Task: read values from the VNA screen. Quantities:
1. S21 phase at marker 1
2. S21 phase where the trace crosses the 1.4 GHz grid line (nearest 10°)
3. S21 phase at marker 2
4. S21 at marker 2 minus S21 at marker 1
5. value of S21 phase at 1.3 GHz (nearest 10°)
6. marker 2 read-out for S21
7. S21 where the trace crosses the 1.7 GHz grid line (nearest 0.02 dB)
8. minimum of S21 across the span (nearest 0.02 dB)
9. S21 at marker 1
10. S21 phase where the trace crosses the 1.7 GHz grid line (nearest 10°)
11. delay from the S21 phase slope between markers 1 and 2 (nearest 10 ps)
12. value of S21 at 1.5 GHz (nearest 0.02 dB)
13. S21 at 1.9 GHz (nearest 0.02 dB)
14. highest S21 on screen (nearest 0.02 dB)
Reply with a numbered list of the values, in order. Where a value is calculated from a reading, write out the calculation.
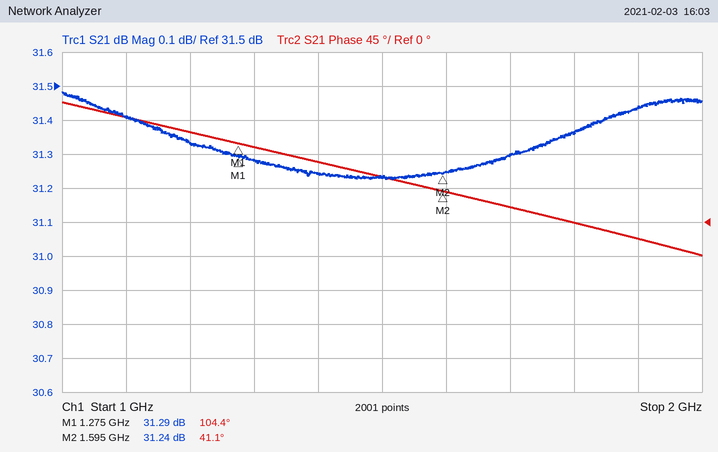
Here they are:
1. 104.4°
2. 80°
3. 41.1°
4. 31.24 − (31.29) = -0.05 dB
5. 100°
6. 31.24 dB
7. 31.30 dB
8. 31.22 dB
9. 31.29 dB
10. 20°
11. −(41.1° − (104.4°))/(360° × 320 MHz) ≈ 549 ps, so 550 ps to the nearest 10 ps
12. 31.24 dB
13. 31.44 dB
14. 31.48 dB
